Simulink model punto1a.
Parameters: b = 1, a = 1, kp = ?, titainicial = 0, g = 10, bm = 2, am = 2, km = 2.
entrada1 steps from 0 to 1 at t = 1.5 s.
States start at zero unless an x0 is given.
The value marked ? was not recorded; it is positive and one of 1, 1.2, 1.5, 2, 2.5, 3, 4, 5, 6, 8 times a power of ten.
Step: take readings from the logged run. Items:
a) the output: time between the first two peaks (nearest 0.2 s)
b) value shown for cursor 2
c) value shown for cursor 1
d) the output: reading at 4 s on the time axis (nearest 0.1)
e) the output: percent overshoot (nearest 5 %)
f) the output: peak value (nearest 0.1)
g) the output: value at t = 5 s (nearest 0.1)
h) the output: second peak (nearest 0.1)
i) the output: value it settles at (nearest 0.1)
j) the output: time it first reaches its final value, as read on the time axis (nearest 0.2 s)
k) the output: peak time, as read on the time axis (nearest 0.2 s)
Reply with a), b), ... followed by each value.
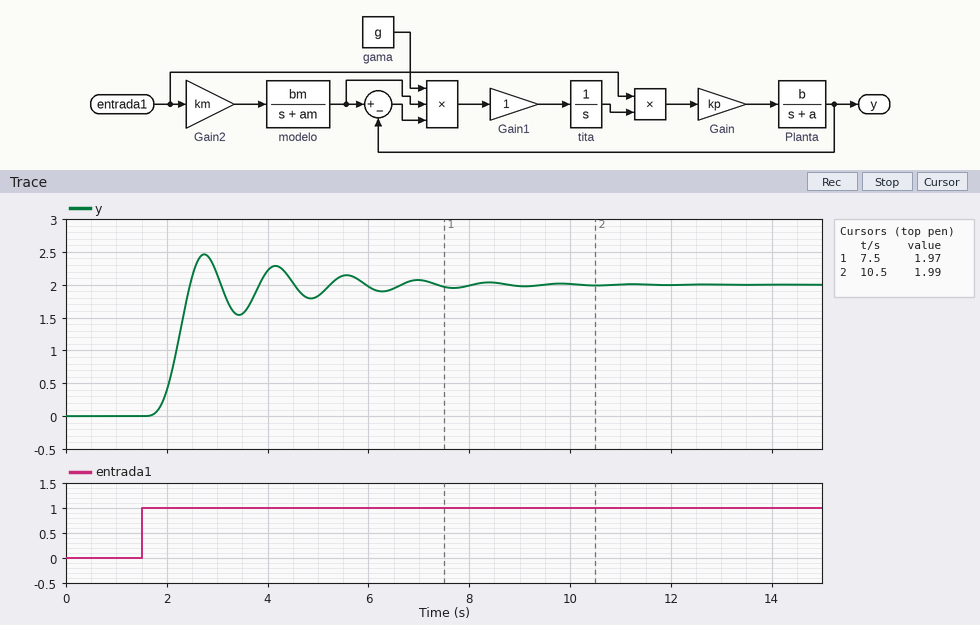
a) 1.4 s
b) 1.99
c) 1.97
d) 2.2
e) 25 %
f) 2.5
g) 1.8
h) 2.3
i) 2.0
j) 2.4 s
k) 2.8 s
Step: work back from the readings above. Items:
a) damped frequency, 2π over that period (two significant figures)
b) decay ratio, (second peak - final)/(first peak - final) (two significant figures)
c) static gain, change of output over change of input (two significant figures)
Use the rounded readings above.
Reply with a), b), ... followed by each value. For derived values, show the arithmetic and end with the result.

a) 2π / 1.4 = 4.5 rad/s
b) (2.3 - 2) / (2.5 - 2) = 0.60
c) (2 - 0) / (1 - 0) = 2.0
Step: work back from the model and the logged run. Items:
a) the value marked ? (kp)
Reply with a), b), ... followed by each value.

a) 1
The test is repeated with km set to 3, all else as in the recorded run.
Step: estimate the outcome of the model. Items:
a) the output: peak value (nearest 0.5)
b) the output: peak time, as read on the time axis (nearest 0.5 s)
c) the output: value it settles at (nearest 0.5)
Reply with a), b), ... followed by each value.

a) 3.5
b) 2.5 s
c) 3.0
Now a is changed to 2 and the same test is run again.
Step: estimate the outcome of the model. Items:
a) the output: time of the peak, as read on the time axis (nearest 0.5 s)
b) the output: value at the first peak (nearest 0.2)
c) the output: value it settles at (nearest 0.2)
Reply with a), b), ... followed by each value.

a) 3.0 s
b) 2.2
c) 2.0
